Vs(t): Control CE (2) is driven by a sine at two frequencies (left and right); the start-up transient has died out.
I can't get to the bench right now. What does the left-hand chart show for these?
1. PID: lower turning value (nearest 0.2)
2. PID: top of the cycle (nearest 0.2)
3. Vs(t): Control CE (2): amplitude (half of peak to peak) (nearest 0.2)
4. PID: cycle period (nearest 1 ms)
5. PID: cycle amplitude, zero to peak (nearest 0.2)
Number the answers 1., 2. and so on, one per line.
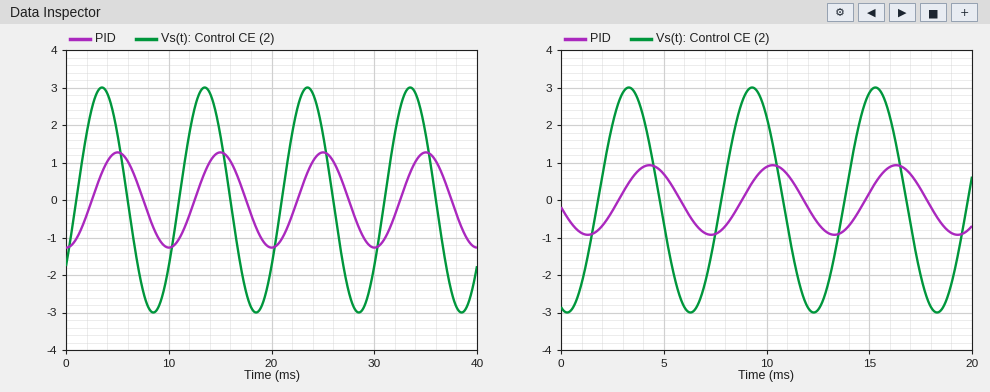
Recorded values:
1. -1.2
2. 1.2
3. 3.0
4. 10 ms
5. 1.2
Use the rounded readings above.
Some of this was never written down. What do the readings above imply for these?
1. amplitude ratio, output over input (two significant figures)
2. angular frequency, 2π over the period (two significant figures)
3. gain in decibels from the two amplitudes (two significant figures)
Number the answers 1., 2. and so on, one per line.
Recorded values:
1. 0.40
2. 0.63 rad/ms
3. -8.0 dB
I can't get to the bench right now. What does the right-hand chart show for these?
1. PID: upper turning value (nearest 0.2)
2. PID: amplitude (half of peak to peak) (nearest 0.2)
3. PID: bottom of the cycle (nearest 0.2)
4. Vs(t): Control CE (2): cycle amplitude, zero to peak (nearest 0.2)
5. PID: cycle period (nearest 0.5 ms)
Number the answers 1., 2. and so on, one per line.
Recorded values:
1. 1.0
2. 1.0
3. -1.0
4. 3.0
5. 6.0 ms
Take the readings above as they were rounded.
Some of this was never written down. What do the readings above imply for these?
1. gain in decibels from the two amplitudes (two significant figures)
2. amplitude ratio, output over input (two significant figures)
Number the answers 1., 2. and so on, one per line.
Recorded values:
1. -9.5 dB
2. 0.33
